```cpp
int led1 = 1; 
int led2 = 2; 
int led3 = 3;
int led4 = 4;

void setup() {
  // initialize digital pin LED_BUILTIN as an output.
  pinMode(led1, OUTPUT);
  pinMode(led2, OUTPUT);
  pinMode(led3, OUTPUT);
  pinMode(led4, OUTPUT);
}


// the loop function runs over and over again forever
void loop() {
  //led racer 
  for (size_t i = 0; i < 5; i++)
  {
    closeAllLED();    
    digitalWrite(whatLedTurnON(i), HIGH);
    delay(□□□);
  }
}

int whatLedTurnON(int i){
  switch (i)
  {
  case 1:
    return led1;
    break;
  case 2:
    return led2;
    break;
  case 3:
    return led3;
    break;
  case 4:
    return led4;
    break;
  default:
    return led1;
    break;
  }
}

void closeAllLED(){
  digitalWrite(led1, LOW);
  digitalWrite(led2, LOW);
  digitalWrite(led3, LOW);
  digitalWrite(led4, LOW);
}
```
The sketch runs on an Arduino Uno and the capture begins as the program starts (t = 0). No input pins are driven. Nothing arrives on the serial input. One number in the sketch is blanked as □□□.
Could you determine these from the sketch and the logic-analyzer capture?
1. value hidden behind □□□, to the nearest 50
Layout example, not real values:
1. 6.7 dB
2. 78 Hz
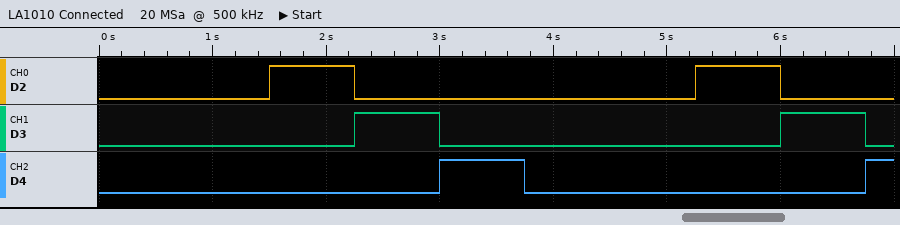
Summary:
1. 750
